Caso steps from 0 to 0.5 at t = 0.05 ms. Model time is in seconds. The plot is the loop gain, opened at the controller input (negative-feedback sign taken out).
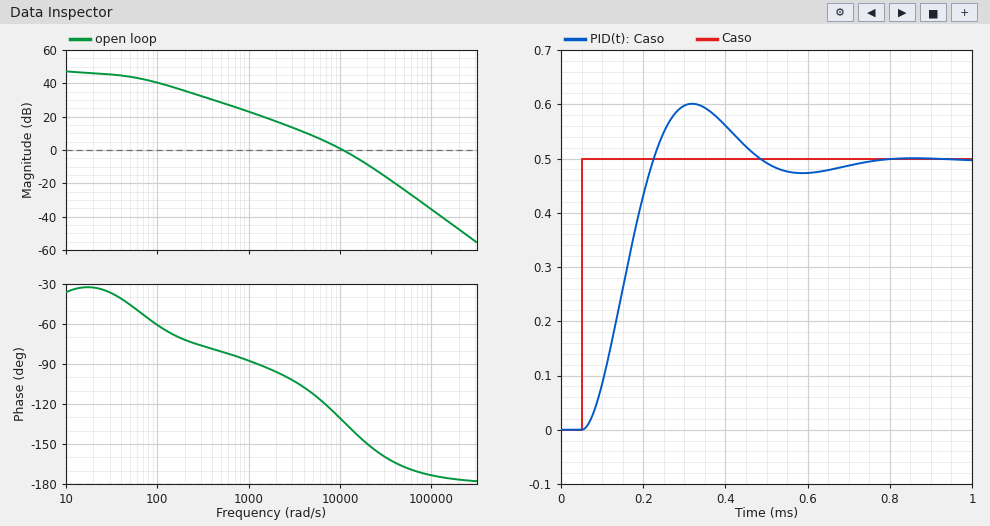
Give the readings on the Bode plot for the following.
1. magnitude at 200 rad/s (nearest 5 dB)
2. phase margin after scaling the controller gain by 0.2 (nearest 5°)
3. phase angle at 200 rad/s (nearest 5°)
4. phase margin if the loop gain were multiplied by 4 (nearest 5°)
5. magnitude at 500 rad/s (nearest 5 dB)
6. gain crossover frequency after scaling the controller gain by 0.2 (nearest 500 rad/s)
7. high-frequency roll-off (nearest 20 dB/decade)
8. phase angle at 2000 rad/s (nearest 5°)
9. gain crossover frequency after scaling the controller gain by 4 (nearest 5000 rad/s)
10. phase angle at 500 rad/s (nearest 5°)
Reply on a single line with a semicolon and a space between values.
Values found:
35 dB; 80°; -70°; 25°; 30 dB; 3000 rad/s; -40 dB/decade; -95°; 25000 rad/s; -80°
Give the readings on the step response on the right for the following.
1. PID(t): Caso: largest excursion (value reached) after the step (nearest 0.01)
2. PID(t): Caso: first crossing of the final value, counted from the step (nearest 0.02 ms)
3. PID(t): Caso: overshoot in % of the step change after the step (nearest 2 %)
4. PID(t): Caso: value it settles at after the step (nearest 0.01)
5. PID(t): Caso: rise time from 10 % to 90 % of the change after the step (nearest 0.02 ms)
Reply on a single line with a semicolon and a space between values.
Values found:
0.60; 0.18 ms; 20 %; 0.50; 0.12 ms
